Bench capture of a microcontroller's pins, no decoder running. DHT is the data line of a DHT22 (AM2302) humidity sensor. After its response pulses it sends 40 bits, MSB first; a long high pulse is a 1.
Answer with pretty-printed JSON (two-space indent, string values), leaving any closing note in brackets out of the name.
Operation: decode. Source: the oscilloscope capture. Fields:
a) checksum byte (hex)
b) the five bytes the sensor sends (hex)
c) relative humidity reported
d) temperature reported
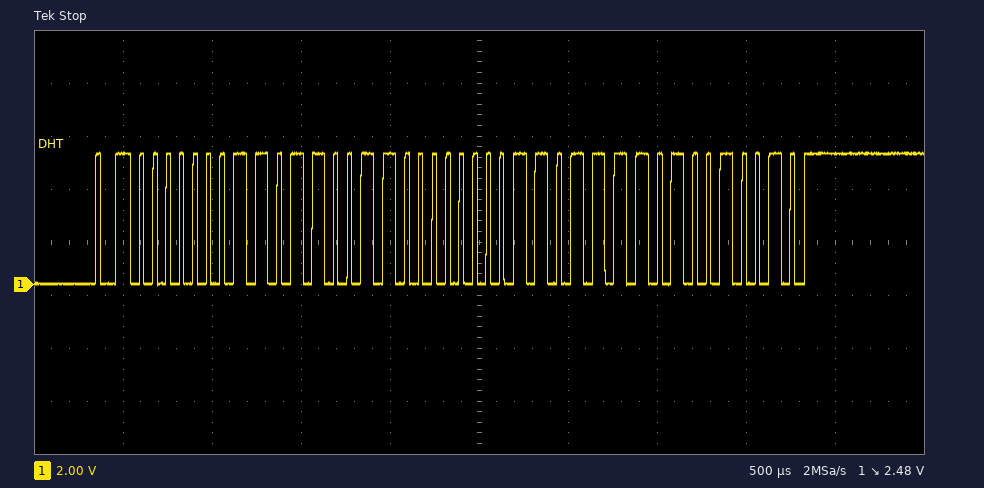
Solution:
{
  "checksum byte": "0x92",
  "the five bytes the sensor sends": "01 B3 00 DE 92",
  "relative humidity reported": "43.5 %",
  "temperature reported": "22.2 °C"
}
